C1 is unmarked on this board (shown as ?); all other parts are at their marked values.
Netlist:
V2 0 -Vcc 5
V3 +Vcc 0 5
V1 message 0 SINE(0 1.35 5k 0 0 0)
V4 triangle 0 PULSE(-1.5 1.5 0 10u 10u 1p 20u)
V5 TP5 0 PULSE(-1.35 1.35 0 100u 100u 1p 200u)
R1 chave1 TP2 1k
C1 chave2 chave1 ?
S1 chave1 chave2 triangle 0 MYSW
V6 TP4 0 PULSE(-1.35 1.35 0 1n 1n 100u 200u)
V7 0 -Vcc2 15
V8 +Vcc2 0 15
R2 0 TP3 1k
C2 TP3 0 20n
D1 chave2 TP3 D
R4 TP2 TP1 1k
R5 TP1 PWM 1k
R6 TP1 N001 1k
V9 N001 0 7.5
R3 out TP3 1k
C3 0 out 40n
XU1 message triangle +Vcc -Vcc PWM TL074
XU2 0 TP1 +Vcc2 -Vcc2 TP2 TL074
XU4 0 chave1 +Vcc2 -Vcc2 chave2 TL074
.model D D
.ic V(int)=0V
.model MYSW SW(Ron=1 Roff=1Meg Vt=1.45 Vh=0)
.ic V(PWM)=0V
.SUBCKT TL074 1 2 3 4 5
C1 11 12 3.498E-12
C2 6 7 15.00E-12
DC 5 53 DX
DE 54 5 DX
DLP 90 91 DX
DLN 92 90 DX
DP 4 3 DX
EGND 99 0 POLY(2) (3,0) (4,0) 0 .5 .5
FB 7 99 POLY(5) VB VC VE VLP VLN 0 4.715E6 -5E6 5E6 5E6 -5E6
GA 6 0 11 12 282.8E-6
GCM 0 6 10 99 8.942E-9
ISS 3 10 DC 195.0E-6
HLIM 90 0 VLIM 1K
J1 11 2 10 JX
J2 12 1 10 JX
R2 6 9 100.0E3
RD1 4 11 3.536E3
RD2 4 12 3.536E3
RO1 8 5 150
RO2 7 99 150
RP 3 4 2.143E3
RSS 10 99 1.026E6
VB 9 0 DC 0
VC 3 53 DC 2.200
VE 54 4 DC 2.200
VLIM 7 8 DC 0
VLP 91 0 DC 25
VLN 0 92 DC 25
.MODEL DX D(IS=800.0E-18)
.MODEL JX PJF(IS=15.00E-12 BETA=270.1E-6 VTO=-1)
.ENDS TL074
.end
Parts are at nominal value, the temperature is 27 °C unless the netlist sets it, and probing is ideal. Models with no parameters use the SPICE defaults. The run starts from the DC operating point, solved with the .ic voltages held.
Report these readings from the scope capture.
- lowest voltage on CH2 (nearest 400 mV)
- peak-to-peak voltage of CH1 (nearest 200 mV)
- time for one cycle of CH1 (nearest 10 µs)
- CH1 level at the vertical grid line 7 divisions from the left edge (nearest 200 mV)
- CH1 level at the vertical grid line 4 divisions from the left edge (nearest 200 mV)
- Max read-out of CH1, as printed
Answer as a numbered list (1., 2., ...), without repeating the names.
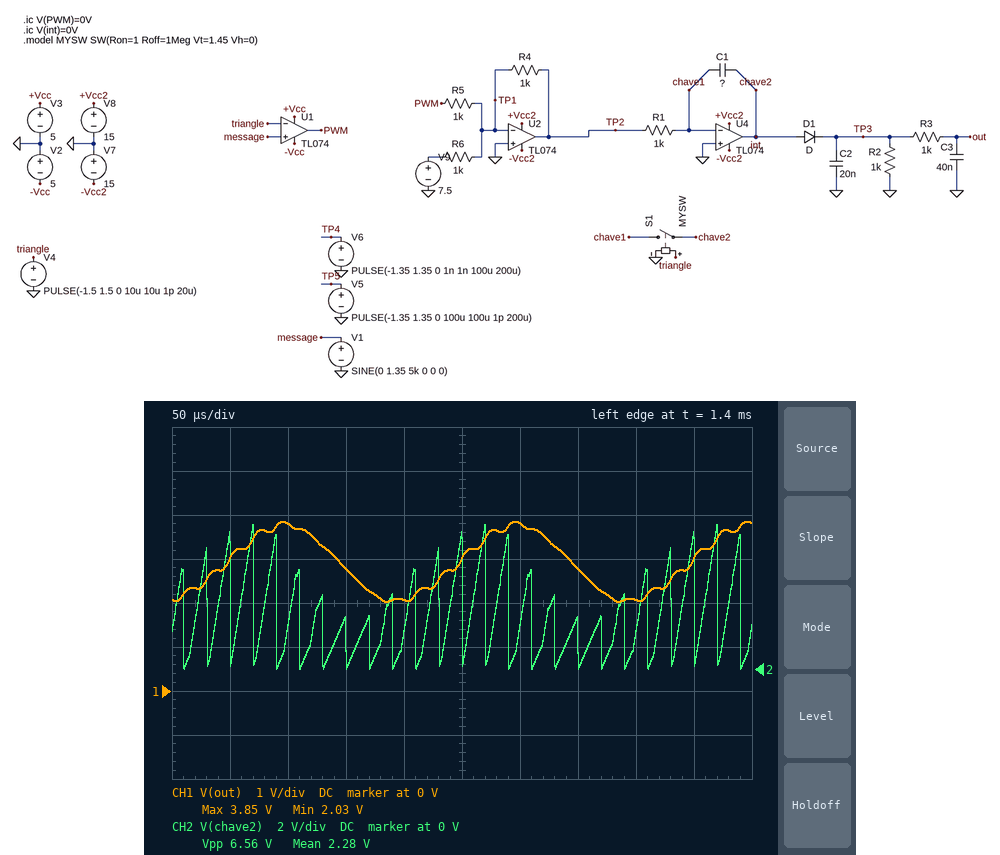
1. 0 V
2. 1.8 V
3. 200 µs
4. 2.8 V
5. 2.0 V
6. 3.85 V
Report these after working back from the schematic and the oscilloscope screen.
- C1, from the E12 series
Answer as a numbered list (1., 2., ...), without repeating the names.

1. 33 nF
